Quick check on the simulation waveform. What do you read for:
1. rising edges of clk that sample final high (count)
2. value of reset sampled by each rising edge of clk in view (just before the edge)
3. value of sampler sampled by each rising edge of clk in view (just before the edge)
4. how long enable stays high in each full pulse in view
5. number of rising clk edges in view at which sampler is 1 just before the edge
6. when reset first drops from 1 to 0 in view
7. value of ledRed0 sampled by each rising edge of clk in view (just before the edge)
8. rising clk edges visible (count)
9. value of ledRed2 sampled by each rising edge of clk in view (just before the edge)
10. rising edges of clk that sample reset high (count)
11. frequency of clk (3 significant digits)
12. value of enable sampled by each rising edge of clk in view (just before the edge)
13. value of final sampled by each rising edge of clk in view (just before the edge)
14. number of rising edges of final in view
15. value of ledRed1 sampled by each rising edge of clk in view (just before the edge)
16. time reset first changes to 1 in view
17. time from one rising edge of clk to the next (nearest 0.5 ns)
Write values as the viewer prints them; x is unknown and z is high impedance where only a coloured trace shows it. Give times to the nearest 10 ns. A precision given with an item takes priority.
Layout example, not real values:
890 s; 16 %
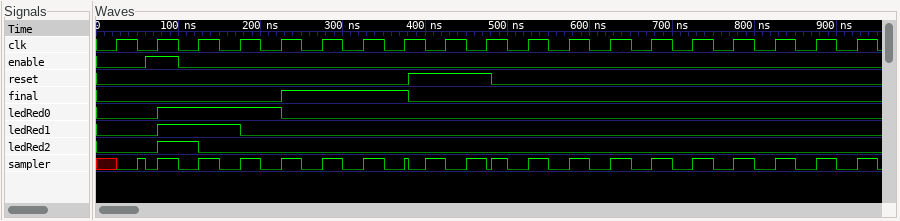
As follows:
3; 0 0 0 0 0 0 0 0 1 1 0 0 0 0 0 0 0 0 0; x 0 0 0 0 0 0 0 1 1 0 0 0 0 0 0 0 0 0; 40 ns; 2; 480 ns; 0 0 1 1 1 0 0 0 0 0 0 0 0 0 0 0 0 0 0; 19; 0 0 1 0 0 0 0 0 0 0 0 0 0 0 0 0 0 0 0; 2; 20.0 MHz; 0 1 0 0 0 0 0 0 0 0 0 0 0 0 0 0 0 0 0; 0 0 0 0 0 1 1 1 0 0 0 0 0 0 0 0 0 0 0; 1; 0 0 1 1 0 0 0 0 0 0 0 0 0 0 0 0 0 0 0; 380 ns; 50 ns
